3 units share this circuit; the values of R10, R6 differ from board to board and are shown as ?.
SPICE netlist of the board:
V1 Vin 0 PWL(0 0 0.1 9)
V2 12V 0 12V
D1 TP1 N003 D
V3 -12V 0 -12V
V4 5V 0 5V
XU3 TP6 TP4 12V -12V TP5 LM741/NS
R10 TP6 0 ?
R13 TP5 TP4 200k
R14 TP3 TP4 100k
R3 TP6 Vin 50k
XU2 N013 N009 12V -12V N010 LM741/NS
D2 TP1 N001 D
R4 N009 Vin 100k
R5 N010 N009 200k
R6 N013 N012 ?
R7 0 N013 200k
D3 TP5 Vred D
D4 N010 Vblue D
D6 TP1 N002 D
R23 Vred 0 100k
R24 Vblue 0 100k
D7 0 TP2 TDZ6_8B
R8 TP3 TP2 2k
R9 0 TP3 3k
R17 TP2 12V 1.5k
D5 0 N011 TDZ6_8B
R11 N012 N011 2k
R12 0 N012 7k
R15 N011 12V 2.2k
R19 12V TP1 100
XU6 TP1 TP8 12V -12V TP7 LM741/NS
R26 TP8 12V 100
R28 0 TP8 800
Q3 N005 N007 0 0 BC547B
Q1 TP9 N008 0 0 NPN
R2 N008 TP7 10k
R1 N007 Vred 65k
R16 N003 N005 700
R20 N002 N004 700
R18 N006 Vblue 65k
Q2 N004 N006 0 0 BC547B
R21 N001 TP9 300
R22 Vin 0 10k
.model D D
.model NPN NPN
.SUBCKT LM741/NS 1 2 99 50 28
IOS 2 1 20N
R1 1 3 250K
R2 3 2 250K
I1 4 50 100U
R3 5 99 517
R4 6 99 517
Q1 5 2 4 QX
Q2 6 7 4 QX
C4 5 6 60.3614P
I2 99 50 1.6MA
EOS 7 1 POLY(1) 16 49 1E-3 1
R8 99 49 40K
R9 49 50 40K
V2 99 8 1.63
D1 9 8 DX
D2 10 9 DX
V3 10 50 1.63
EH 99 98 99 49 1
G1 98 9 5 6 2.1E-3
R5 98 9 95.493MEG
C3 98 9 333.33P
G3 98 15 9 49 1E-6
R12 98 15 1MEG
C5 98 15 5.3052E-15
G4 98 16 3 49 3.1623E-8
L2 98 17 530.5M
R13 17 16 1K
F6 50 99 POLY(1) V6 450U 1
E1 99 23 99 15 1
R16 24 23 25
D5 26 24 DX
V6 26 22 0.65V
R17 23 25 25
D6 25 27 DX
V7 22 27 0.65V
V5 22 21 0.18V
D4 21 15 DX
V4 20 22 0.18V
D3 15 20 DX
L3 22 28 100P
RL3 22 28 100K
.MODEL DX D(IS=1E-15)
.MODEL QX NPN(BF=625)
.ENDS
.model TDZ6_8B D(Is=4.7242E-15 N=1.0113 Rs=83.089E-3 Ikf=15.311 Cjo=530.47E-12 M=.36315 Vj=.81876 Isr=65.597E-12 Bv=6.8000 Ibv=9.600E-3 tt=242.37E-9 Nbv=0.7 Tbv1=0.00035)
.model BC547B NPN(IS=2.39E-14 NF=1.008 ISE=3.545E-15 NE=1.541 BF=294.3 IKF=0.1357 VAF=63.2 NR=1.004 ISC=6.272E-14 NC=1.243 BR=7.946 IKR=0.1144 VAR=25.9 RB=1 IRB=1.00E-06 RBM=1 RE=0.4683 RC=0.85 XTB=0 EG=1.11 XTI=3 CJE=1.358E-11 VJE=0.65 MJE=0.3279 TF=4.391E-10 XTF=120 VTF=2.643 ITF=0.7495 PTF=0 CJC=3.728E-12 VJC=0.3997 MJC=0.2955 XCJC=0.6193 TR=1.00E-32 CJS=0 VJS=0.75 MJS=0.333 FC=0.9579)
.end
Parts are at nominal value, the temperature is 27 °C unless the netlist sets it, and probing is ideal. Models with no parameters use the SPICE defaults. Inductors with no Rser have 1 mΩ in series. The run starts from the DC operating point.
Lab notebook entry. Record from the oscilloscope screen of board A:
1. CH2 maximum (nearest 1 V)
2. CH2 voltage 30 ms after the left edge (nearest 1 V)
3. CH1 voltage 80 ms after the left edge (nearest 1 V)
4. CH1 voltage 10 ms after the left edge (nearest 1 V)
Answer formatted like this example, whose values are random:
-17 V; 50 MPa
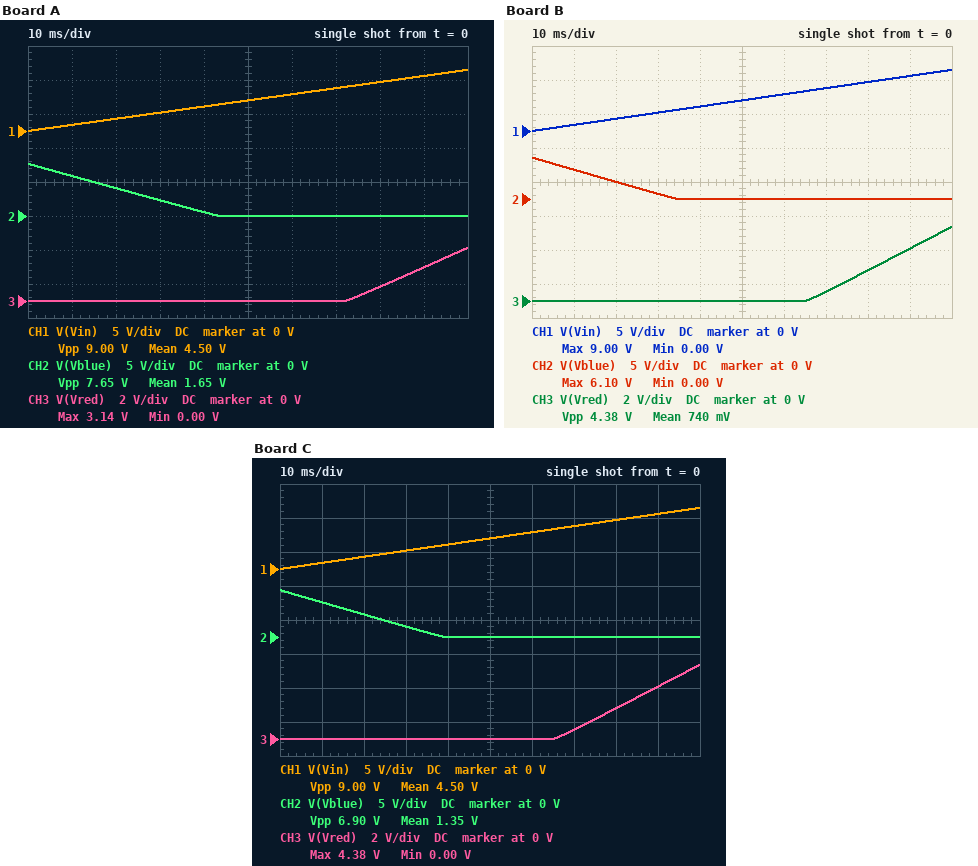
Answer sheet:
8 V; 2 V; 7 V; 1 V
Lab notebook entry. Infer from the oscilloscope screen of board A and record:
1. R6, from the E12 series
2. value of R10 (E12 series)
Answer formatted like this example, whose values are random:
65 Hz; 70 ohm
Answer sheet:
180 kΩ; 39 kΩ
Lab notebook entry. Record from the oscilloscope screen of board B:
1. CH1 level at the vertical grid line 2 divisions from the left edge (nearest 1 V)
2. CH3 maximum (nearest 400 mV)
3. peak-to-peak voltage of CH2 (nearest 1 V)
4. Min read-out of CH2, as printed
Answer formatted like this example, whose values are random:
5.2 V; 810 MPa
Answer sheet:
2 V; 4.4 V; 6 V; 0.00 V
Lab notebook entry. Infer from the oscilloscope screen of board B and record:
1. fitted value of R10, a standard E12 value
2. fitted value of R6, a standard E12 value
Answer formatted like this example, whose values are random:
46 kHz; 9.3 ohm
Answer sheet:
47 kΩ; 270 kΩ
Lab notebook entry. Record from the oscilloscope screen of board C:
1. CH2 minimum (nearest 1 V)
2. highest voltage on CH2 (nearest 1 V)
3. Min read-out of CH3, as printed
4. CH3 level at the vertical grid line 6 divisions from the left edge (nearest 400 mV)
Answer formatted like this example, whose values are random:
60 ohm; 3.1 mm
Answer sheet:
0 V; 7 V; 0.00 V; 0 V
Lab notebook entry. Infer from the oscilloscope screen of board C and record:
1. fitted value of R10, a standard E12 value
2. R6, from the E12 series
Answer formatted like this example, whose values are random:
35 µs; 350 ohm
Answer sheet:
47 kΩ; 220 kΩ
